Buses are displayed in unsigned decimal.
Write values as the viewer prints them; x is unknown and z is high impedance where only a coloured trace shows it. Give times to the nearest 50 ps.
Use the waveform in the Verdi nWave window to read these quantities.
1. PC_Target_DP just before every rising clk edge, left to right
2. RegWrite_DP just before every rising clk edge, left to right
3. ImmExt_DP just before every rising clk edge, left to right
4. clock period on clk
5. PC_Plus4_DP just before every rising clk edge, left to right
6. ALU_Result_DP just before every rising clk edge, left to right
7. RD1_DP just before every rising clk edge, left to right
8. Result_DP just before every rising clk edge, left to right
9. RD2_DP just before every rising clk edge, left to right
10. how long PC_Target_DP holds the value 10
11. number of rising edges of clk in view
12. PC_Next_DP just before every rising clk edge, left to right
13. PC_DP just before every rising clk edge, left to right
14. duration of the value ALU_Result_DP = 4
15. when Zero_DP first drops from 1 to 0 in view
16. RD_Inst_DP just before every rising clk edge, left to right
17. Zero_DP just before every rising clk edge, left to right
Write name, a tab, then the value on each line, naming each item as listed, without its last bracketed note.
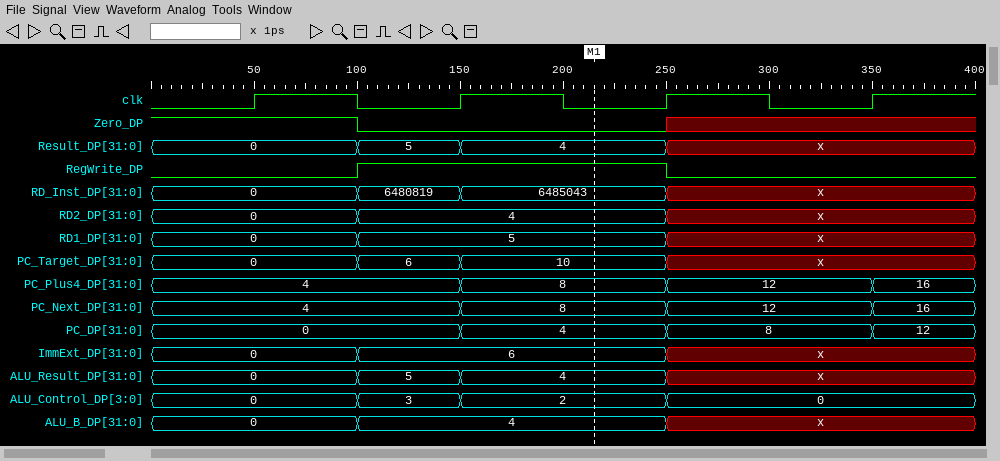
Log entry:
PC_Target_DP just before every rising clk edge, left to right	0, 6, 10, x
RegWrite_DP just before every rising clk edge, left to right	0 1 1 0
ImmExt_DP just before every rising clk edge, left to right	0, 6, 6, x
clock period on clk	100 ps
PC_Plus4_DP just before every rising clk edge, left to right	4, 4, 8, 12
ALU_Result_DP just before every rising clk edge, left to right	0, 5, 4, x
RD1_DP just before every rising clk edge, left to right	0, 5, 5, x
Result_DP just before every rising clk edge, left to right	0, 5, 4, x
RD2_DP just before every rising clk edge, left to right	0, 4, 4, x
how long PC_Target_DP holds the value 10	100 ps
number of rising edges of clk in view	4
PC_Next_DP just before every rising clk edge, left to right	4, 4, 8, 12
PC_DP just before every rising clk edge, left to right	0, 0, 4, 8
duration of the value ALU_Result_DP = 4	100 ps
when Zero_DP first drops from 1 to 0 in view	100 ps
RD_Inst_DP just before every rising clk edge, left to right	0, 6480819, 6485043, x
Zero_DP just before every rising clk edge, left to right	1 0 0 x
